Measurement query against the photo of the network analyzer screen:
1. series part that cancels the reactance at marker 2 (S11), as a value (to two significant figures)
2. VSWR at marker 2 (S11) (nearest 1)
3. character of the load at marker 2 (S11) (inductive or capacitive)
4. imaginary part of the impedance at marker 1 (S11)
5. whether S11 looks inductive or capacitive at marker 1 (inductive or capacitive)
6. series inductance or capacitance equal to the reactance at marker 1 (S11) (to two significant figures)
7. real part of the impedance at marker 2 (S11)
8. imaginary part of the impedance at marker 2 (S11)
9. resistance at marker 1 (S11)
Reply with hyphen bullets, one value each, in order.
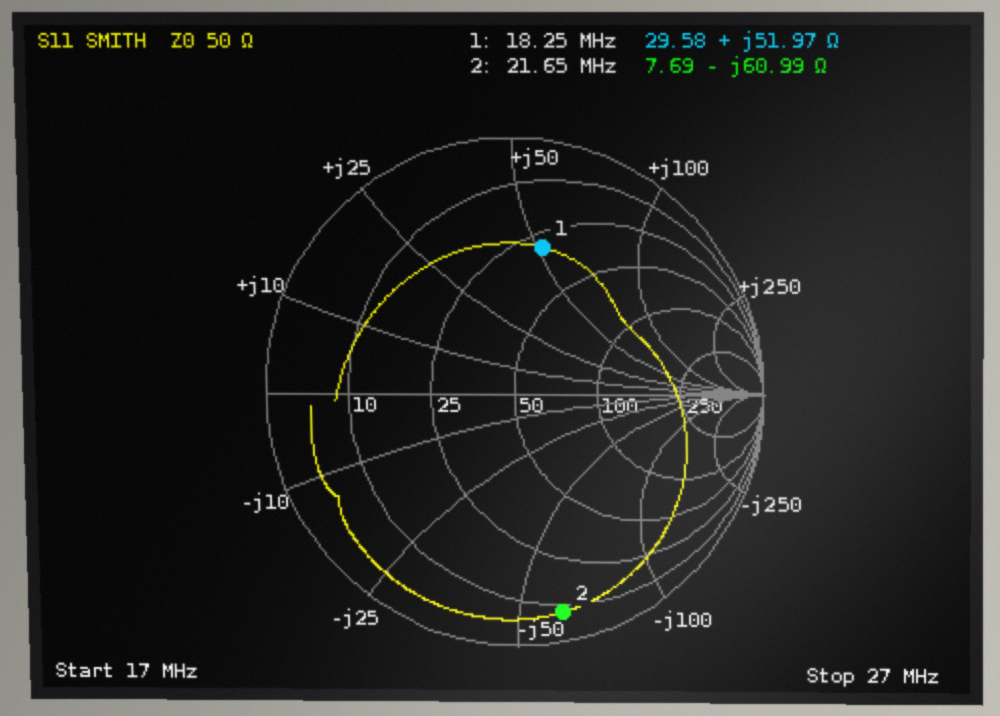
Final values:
- 450 nH
- 16
- capacitive
- +51.97 Ω
- inductive
- 450 nH
- 7.69 Ω
- -60.99 Ω
- 29.58 Ω
